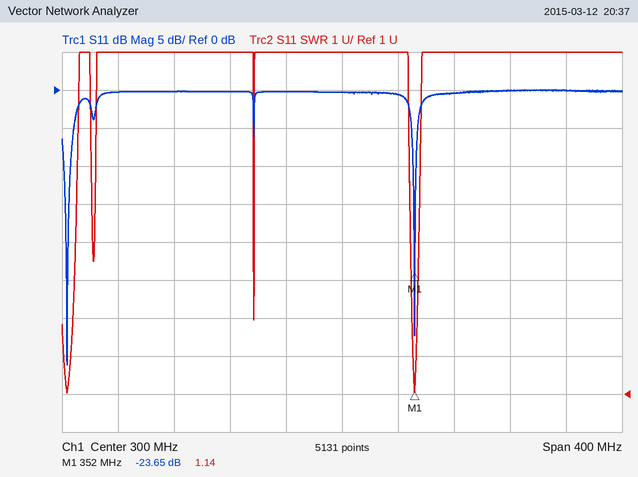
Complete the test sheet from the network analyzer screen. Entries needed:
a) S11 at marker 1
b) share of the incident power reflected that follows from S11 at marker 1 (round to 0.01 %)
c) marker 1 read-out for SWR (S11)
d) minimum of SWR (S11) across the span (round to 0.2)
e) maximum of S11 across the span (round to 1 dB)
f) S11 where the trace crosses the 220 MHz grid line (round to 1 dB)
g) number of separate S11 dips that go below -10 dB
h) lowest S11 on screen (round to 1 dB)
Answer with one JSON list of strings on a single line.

["-23.65 dB", "0.43 %", "1.14", "1.0", "0 dB", "0 dB", "2", "-36 dB"]
